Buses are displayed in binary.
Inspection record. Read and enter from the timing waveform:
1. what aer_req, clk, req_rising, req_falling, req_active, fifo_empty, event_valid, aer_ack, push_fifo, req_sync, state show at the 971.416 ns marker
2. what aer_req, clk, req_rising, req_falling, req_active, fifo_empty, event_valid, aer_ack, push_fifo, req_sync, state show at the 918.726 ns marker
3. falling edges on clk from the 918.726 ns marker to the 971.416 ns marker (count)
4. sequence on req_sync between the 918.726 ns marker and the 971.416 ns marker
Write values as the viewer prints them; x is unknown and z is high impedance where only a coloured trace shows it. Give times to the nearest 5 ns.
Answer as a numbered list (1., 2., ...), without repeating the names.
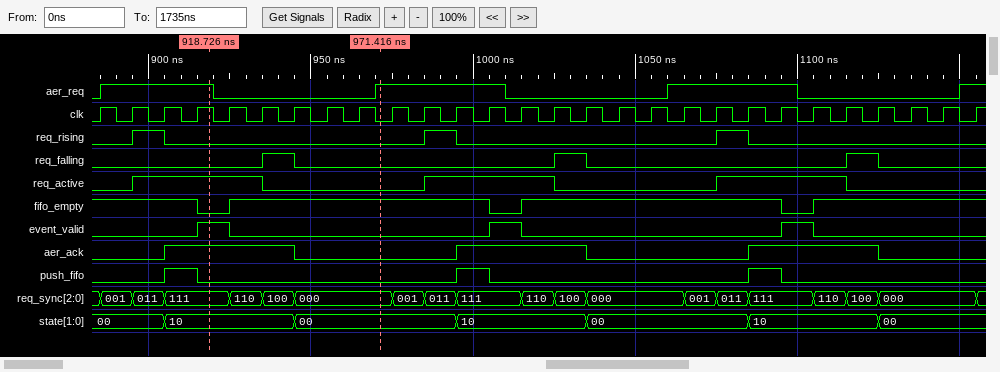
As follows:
1. aer_req=1, clk=0, req_rising=0, req_falling=0, req_active=0, fifo_empty=1, event_valid=0, aer_ack=0, push_fifo=0, req_sync=000, state=00
2. aer_req=1, clk=1, req_rising=0, req_falling=0, req_active=1, fifo_empty=0, event_valid=1, aer_ack=1, push_fifo=0, req_sync=111, state=10
3. 6
4. 111, 110, 100, 000
